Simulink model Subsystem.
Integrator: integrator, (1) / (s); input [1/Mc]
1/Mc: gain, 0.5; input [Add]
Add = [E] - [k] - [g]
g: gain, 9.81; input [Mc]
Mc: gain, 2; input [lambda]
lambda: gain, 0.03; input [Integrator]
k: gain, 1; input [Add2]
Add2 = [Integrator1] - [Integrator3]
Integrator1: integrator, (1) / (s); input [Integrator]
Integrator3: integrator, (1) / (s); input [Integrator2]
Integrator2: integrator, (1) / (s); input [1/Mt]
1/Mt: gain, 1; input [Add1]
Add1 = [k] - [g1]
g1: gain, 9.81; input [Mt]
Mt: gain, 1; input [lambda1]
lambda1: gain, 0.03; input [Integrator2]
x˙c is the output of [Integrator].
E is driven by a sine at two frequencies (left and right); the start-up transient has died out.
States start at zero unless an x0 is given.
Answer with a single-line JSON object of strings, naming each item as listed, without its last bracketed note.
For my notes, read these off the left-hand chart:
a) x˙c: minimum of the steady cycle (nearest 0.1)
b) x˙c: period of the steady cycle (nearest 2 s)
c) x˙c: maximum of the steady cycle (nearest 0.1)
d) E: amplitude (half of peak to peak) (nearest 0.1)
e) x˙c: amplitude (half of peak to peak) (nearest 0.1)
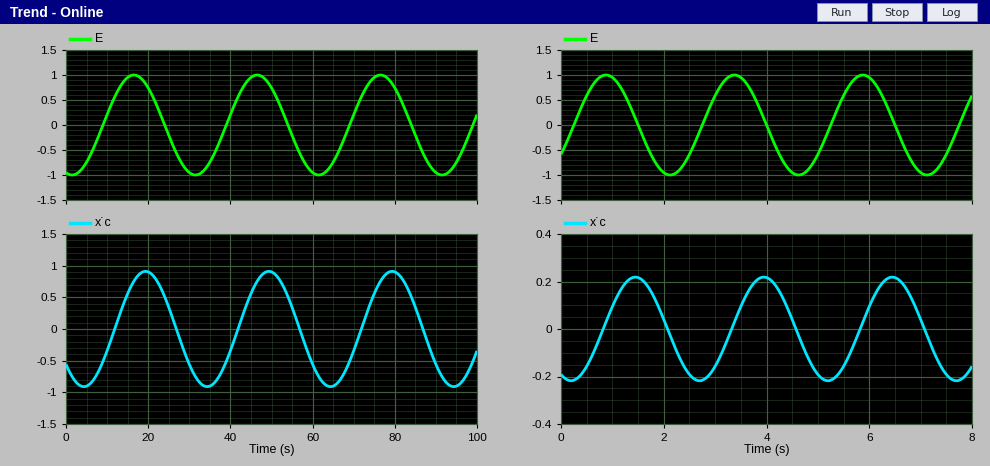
{"x˙c: minimum of the steady cycle": "-0.9", "x˙c: period of the steady cycle": "30 s", "x˙c: maximum of the steady cycle": "0.9", "E: amplitude (half of peak to peak)": "1.0", "x˙c: amplitude (half of peak to peak)": "0.9"}
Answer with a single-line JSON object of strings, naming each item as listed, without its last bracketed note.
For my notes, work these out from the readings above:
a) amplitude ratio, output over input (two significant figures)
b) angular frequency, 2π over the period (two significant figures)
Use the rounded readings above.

{"amplitude ratio, output over input": "0.90", "angular frequency, 2π over the period": "0.21 rad/s"}
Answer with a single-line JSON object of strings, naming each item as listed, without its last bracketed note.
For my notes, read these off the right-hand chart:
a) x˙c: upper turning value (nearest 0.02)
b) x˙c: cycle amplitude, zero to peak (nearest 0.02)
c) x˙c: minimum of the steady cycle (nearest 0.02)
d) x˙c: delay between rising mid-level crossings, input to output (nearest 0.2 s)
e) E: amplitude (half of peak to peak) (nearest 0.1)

{"x˙c: upper turning value": "0.22", "x˙c: cycle amplitude, zero to peak": "0.22", "x˙c: minimum of the steady cycle": "-0.22", "x˙c: delay between rising mid-level crossings, input to output": "0.6 s", "E: amplitude (half of peak to peak)": "1.0"}
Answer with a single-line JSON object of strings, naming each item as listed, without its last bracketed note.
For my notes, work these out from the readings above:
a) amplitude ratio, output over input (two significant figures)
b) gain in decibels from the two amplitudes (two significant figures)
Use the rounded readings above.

{"amplitude ratio, output over input": "0.22", "gain in decibels from the two amplitudes": "-13 dB"}
